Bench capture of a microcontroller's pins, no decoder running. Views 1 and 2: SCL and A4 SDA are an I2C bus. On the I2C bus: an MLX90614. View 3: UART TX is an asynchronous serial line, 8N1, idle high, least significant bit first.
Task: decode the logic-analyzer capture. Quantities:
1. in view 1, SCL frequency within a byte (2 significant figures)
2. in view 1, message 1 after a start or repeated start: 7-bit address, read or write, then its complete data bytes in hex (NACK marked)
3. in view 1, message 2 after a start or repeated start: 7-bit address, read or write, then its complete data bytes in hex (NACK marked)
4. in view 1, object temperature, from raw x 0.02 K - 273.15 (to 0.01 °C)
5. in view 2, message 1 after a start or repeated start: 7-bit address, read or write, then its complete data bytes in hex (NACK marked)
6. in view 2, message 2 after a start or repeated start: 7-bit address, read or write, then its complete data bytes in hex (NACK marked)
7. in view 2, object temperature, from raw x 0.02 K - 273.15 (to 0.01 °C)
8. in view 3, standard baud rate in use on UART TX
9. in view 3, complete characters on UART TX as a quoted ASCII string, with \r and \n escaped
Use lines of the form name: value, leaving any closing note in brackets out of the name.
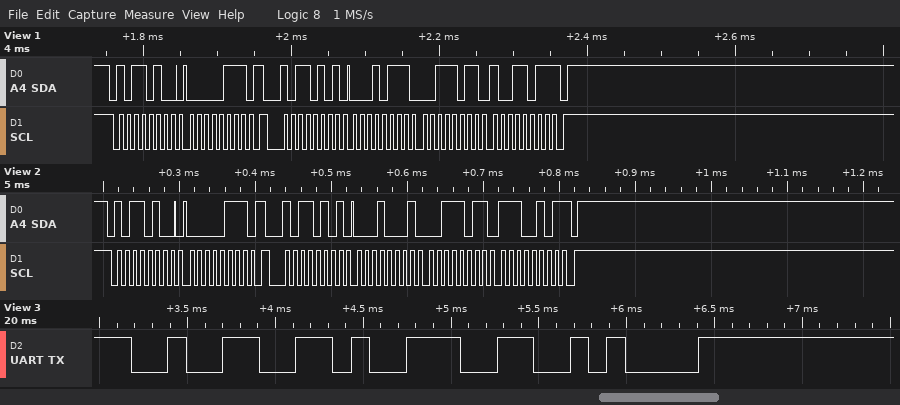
in view 1, SCL frequency within a byte: 100 kHz
in view 1, message 1 after a start or repeated start: 7-bit address, read or write, then its complete data bytes in hex: 0x5A write: 07
in view 1, message 2 after a start or repeated start: 7-bit address, read or write, then its complete data bytes in hex: 0x5A read: 17 3B 9B NACK
in view 1, object temperature, from raw x 0.02 K - 273.15: 29.39 °C
in view 2, message 1 after a start or repeated start: 7-bit address, read or write, then its complete data bytes in hex: 0x5A write: 07
in view 2, message 2 after a start or repeated start: 7-bit address, read or write, then its complete data bytes in hex: 0x5A read: 11 3B E5 NACK
in view 2, object temperature, from raw x 0.02 K - 273.15: 29.27 °C
in view 3, standard baud rate in use on UART TX: 9600 baud
in view 3, complete characters on UART TX as a quoted ASCII string, with \r and \n escaped: "29\n"
